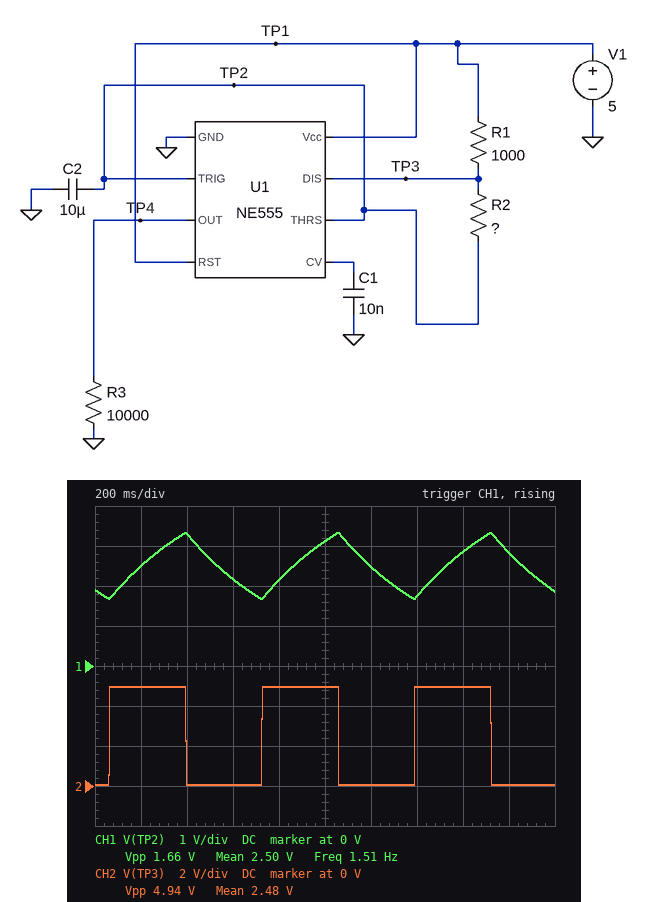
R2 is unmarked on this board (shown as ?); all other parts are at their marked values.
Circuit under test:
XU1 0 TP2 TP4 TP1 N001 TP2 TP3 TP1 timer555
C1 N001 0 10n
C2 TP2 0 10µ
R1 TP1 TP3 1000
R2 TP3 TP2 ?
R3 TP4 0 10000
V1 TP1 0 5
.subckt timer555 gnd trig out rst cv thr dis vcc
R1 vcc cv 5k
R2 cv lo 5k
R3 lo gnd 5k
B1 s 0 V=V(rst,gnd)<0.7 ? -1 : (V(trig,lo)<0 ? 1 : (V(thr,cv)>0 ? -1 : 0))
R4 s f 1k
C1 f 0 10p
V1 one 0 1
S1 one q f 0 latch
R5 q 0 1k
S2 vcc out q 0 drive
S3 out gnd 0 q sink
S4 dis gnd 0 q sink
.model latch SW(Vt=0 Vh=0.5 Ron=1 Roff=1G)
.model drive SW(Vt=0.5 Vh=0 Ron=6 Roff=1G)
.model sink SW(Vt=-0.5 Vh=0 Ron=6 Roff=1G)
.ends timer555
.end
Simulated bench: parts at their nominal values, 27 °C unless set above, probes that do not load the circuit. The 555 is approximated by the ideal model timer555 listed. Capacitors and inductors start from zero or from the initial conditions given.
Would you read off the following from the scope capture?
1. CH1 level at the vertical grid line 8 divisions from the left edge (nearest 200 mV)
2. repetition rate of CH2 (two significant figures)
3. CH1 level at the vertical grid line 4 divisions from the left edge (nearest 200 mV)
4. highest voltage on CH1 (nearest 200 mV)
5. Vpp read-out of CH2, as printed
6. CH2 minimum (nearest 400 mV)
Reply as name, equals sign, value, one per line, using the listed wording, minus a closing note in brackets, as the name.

CH1 level at the vertical grid line 8 divisions from the left edge = 2.8 V
repetition rate of CH2 = 1.5 Hz
CH1 level at the vertical grid line 4 divisions from the left edge = 2.2 V
highest voltage on CH1 = 3.4 V
Vpp read-out of CH2, as printed = 4.94 V
CH2 minimum = 0 V
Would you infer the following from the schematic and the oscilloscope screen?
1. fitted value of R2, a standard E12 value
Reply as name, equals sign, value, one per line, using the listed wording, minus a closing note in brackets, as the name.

fitted value of R2, a standard E12 value = 47 kΩ
